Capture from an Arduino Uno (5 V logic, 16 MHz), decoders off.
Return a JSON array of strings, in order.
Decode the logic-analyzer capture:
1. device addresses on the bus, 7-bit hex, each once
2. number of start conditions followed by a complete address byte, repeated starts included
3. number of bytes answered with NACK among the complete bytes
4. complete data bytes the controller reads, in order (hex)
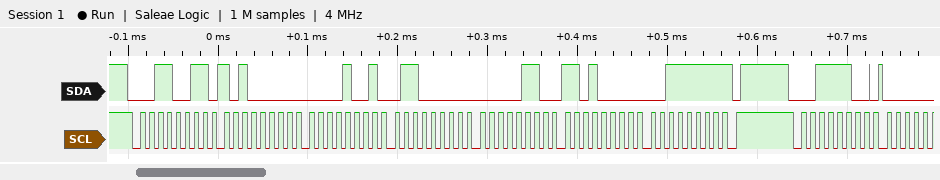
["0x19 0x1E", "2", "1", "A0 09 60 06 D0 3F"]
